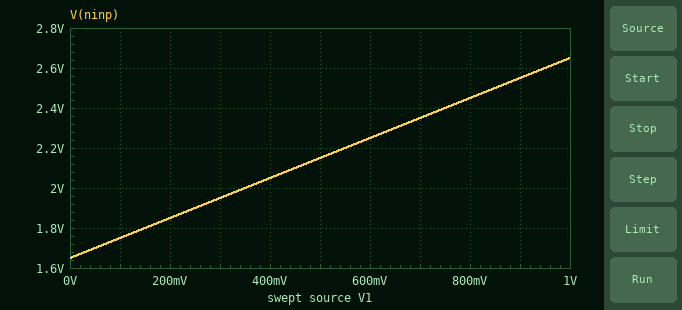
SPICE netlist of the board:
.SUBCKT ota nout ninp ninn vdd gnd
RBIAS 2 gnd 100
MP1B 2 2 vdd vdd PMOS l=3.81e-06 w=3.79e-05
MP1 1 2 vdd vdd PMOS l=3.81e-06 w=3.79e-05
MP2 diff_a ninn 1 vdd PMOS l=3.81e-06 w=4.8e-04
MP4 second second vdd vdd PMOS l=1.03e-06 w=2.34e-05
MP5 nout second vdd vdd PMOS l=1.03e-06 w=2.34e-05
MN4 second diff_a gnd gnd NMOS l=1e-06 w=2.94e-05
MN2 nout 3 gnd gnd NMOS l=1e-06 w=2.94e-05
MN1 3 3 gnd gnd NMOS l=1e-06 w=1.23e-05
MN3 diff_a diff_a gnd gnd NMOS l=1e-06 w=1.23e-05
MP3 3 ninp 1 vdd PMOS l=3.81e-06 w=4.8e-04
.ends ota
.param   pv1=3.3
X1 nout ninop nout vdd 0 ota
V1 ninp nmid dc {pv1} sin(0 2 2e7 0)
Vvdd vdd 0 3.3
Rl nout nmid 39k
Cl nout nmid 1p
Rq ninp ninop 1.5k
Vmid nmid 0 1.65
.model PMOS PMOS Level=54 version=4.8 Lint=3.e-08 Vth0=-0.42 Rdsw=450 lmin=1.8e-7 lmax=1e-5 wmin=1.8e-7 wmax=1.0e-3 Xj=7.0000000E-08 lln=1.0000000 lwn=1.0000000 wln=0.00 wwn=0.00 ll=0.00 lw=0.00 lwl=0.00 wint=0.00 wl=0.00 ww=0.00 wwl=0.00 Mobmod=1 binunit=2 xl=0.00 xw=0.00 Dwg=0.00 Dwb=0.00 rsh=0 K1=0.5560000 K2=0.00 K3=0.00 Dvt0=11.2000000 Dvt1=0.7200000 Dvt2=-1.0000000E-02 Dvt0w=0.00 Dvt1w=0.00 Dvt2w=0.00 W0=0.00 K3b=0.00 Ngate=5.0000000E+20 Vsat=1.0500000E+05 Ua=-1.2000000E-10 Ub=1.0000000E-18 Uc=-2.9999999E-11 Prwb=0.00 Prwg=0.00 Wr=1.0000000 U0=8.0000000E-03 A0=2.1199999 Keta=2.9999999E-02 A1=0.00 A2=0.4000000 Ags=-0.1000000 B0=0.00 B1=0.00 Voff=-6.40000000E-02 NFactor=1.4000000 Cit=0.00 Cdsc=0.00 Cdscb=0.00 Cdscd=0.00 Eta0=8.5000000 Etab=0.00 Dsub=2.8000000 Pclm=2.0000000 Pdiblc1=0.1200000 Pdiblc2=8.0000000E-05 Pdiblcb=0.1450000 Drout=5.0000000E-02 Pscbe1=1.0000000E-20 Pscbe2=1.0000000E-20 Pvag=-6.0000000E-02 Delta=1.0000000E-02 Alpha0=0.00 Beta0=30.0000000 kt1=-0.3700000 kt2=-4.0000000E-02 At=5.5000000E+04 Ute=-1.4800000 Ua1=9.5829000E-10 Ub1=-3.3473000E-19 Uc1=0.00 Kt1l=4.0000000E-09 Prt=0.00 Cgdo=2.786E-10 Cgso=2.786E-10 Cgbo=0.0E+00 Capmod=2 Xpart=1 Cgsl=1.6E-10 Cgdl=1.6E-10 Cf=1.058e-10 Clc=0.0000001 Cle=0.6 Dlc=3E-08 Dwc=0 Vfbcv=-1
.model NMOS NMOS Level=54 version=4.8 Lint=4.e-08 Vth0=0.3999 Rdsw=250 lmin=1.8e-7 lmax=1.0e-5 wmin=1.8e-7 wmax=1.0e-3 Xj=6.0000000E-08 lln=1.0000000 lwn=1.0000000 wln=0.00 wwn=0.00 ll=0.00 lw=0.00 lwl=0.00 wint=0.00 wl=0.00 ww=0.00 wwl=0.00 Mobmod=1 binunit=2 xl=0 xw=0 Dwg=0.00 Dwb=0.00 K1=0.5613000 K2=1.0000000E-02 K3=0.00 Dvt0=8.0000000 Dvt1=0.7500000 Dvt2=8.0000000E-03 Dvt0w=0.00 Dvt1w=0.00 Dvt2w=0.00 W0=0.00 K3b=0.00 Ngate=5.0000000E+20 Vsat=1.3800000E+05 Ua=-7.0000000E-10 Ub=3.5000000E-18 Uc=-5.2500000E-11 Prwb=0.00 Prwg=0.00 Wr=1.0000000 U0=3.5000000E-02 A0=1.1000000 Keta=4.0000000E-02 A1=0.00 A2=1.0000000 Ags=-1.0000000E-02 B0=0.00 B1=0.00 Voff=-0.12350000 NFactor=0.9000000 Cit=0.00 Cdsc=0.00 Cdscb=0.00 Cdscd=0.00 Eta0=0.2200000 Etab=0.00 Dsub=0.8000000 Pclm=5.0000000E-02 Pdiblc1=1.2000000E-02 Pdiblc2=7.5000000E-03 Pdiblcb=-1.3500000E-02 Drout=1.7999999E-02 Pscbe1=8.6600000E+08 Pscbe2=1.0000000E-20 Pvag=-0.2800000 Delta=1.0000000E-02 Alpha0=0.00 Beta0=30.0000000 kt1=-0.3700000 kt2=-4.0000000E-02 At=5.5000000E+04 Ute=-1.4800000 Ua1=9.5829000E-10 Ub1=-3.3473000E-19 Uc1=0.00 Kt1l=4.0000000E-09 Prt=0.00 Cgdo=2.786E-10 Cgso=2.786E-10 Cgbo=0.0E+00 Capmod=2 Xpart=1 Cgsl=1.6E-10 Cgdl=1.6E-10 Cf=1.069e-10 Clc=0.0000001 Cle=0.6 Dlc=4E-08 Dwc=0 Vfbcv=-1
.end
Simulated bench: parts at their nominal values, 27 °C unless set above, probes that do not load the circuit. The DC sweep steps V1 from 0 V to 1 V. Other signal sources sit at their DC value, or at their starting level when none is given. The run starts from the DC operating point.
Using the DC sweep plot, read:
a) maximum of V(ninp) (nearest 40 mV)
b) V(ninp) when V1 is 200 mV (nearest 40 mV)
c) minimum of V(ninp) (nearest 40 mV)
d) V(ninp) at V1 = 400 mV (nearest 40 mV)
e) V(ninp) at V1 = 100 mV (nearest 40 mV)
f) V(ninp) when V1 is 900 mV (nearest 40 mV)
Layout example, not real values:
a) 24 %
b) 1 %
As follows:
a) 2.64 V
b) 1.84 V
c) 1.64 V
d) 2.04 V
e) 1.76 V
f) 2.56 V
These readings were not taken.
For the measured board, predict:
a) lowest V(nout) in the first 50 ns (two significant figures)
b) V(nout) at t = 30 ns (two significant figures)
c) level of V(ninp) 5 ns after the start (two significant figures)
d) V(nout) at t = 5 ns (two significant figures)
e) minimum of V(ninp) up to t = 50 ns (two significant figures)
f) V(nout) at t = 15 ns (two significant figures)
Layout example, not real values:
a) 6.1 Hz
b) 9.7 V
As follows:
a) 110 mV
b) 2.6 V
c) 2.8 V
d) 1.8 V
e) -350 mV
f) 2.7 V
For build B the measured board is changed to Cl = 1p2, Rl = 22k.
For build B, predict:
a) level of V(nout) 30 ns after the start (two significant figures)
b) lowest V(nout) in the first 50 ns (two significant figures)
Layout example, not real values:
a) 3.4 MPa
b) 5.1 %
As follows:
a) 2.5 V
b) 120 mV
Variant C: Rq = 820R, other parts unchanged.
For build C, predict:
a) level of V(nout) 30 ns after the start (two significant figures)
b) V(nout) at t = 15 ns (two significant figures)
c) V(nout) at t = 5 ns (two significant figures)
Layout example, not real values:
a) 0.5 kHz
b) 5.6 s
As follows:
a) 2.4 V
b) 2.8 V
c) 1.9 V
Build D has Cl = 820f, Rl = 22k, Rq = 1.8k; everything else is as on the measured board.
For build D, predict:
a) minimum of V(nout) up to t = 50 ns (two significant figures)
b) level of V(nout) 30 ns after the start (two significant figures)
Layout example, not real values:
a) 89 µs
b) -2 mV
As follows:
a) 150 mV
b) 2.5 V
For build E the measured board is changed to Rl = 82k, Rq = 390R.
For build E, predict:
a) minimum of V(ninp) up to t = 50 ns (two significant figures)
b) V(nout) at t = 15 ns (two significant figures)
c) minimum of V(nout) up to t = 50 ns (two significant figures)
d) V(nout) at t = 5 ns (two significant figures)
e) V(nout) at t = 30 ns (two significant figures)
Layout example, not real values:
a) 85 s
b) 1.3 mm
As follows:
a) -350 mV
b) 2.8 V
c) 95 mV
d) 2.1 V
e) 2.0 V
